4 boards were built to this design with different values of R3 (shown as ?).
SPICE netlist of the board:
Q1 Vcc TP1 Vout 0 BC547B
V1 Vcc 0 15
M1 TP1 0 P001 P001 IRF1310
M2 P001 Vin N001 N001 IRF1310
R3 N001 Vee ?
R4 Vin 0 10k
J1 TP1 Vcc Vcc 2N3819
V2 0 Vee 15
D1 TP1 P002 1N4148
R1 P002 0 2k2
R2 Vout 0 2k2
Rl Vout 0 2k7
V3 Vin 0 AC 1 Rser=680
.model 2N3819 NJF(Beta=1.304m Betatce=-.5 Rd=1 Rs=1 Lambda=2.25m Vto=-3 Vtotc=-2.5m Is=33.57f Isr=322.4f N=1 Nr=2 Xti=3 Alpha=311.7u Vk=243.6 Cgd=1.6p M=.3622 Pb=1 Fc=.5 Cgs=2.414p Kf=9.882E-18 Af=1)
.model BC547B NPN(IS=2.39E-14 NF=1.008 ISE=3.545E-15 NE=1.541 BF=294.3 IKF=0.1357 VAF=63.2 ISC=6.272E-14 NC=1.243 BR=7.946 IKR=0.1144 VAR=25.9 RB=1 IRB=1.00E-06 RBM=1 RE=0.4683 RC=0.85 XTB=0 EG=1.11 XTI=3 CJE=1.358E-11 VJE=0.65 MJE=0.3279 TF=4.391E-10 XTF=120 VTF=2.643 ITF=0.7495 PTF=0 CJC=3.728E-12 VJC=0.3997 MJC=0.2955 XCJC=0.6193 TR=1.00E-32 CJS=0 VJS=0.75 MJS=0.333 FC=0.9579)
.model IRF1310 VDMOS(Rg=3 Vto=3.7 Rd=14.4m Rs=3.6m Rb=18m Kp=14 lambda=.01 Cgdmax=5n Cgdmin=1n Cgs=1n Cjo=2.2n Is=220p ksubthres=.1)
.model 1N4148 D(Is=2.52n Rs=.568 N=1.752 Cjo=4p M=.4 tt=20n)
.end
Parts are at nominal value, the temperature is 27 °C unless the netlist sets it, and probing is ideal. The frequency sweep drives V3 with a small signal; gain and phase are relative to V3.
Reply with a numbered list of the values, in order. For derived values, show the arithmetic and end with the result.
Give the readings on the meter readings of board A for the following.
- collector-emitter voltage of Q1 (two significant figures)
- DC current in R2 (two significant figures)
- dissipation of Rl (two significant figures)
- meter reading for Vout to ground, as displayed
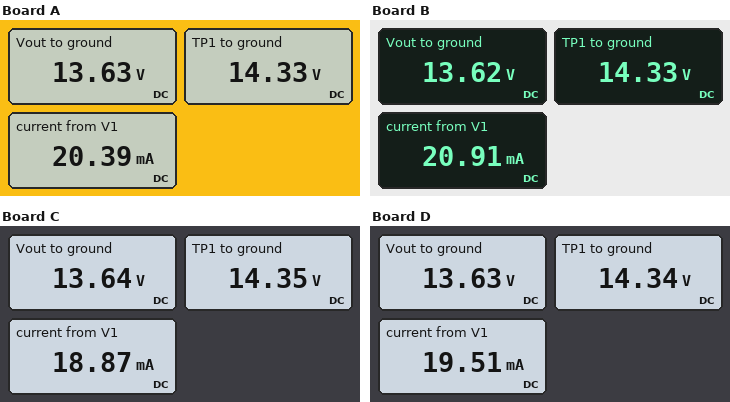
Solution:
1. 15 V - 13.63 V = 1.4 V
2. (13.63 V) / 2.2 kΩ = 6.2 mA
3. (13.63 V)^2 / 2.7 kΩ = 69 mW
4. 13.63 V
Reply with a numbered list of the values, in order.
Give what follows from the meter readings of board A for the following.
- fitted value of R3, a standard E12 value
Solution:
1. 3.9 kΩ
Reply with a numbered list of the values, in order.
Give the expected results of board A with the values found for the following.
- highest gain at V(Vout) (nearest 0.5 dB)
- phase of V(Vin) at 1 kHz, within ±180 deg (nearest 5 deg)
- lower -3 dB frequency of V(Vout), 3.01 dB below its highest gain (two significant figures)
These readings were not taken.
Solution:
1. -39.0 dB
2. 0 deg
3. 42 kHz
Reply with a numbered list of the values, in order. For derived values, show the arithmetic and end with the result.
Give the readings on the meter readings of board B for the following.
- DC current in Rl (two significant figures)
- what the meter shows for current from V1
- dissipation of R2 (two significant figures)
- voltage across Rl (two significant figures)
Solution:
1. (13.62 V) / 2.7 kΩ = 5.0 mA
2. 20.91 mA
3. (13.62 V)^2 / 2.2 kΩ = 84 mW
4. 13.62 V = 14 V
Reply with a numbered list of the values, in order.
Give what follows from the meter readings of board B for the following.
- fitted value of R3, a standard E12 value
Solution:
1. 3.3 kΩ
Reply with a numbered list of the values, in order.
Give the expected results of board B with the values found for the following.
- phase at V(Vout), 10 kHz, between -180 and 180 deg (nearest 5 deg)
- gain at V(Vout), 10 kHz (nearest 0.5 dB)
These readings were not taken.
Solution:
1. 90 deg
2. -52.5 dB
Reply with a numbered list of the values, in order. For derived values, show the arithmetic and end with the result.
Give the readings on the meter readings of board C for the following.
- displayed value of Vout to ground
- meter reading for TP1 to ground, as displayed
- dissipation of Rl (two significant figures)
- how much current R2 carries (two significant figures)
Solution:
1. 13.64 V
2. 14.35 V
3. (13.64 V)^2 / 2.7 kΩ = 69 mW
4. (13.64 V) / 2.2 kΩ = 6.2 mA
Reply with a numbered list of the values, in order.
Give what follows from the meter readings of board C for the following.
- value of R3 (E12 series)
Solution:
1. 8.2 kΩ
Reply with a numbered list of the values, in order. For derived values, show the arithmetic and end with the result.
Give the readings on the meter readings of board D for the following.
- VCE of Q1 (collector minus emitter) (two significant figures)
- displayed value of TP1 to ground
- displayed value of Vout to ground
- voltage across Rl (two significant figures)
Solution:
1. 15 V - 13.63 V = 1.4 V
2. 14.34 V
3. 13.63 V
4. 13.63 V = 14 V
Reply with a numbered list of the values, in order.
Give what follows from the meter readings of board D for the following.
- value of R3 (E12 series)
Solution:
1. 5.6 kΩ
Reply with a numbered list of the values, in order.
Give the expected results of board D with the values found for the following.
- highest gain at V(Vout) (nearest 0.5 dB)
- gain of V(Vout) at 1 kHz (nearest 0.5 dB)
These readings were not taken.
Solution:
1. -37.5 dB
2. -64.5 dB
